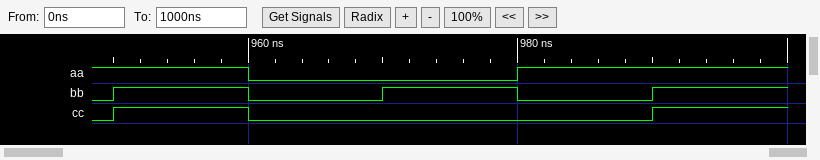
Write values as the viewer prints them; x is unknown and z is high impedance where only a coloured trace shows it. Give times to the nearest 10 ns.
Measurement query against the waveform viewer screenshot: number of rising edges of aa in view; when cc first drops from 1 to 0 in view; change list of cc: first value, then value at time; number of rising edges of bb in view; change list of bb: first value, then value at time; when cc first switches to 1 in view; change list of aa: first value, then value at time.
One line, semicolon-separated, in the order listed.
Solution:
1; 960 ns; 0, 1 at 950 ns, 0 at 960 ns, 1 at 990 ns; 3; 0, 1 at 950 ns, 0 at 960 ns, 1 at 970 ns, 0 at 980 ns, 1 at 990 ns; 950 ns; 1, 0 at 960 ns, 1 at 980 ns
